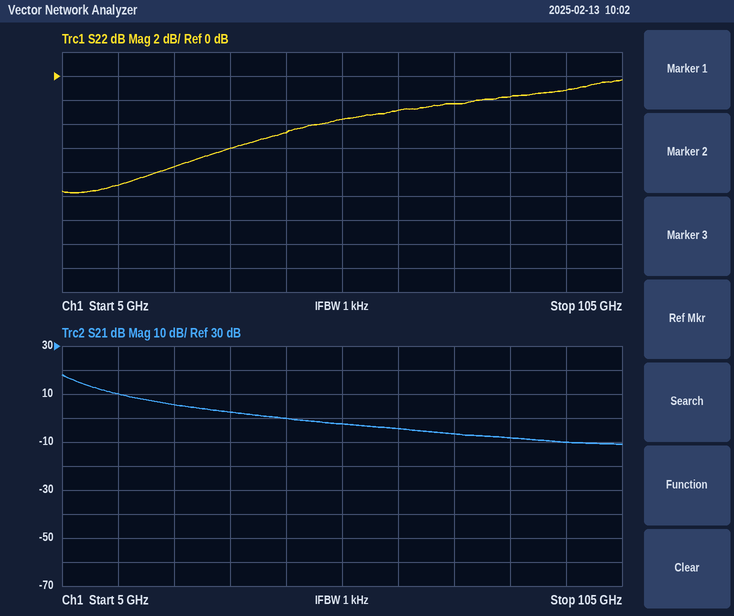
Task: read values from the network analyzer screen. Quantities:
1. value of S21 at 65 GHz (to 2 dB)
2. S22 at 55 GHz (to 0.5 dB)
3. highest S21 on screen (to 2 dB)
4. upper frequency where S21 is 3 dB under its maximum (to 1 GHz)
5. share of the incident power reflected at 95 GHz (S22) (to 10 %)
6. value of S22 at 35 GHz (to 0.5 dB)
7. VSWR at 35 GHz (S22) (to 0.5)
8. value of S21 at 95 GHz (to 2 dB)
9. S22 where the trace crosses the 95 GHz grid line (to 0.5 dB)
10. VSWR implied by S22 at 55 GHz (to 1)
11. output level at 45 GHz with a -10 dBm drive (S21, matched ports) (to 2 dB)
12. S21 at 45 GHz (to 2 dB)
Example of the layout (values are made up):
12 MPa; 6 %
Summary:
-4 dB; -3.5 dB; 18 dB; 8 GHz; 80 %; -6.0 dB; 3.0; -10 dB; -1.0 dB; 5; -10 dBm; 0 dB
